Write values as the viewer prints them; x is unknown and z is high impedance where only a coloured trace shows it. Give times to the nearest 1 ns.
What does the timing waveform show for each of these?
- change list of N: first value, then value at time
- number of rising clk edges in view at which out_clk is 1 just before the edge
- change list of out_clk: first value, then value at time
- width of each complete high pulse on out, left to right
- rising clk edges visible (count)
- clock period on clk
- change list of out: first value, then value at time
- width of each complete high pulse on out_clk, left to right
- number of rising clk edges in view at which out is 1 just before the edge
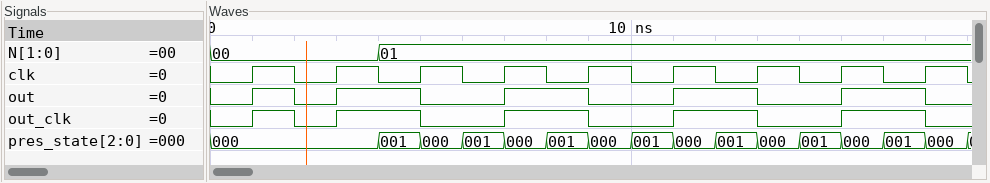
00, 01 at 4 ns
4
0, 1 at 1 ns, 0 at 2 ns, 1 at 3 ns, 0 at 5 ns, 1 at 7 ns, 0 at 9 ns, 1 at 11 ns, 0 at 13 ns, 1 at 15 ns, 0 at 17 ns
1 ns, 2 ns, 2 ns, 2 ns, 2 ns
9
2 ns
0, 1 at 1 ns, 0 at 2 ns, 1 at 3 ns, 0 at 5 ns, 1 at 7 ns, 0 at 9 ns, 1 at 11 ns, 0 at 13 ns, 1 at 15 ns, 0 at 17 ns
1 ns, 2 ns, 2 ns, 2 ns, 2 ns
4
